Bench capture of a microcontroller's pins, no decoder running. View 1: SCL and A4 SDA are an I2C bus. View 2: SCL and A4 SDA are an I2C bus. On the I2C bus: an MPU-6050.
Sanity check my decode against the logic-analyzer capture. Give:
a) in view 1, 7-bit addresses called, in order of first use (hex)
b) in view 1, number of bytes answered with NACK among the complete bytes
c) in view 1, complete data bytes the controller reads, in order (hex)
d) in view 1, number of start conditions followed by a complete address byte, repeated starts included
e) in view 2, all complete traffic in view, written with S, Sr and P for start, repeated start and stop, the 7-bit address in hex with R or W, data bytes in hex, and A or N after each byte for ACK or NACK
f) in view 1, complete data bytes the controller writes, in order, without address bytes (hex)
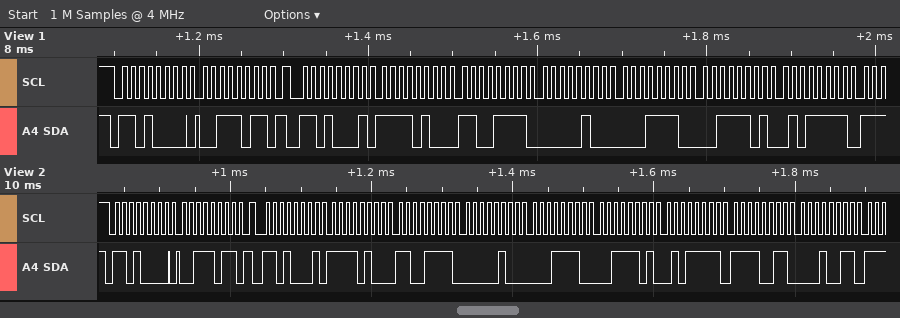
0x68
0
F4 CF 04 1E 3D 5F
2
S 68W A 3B A Sr 68R A F4 A CF A 04 A 1E A 3D A 5F A F3 A 13 A
3B
